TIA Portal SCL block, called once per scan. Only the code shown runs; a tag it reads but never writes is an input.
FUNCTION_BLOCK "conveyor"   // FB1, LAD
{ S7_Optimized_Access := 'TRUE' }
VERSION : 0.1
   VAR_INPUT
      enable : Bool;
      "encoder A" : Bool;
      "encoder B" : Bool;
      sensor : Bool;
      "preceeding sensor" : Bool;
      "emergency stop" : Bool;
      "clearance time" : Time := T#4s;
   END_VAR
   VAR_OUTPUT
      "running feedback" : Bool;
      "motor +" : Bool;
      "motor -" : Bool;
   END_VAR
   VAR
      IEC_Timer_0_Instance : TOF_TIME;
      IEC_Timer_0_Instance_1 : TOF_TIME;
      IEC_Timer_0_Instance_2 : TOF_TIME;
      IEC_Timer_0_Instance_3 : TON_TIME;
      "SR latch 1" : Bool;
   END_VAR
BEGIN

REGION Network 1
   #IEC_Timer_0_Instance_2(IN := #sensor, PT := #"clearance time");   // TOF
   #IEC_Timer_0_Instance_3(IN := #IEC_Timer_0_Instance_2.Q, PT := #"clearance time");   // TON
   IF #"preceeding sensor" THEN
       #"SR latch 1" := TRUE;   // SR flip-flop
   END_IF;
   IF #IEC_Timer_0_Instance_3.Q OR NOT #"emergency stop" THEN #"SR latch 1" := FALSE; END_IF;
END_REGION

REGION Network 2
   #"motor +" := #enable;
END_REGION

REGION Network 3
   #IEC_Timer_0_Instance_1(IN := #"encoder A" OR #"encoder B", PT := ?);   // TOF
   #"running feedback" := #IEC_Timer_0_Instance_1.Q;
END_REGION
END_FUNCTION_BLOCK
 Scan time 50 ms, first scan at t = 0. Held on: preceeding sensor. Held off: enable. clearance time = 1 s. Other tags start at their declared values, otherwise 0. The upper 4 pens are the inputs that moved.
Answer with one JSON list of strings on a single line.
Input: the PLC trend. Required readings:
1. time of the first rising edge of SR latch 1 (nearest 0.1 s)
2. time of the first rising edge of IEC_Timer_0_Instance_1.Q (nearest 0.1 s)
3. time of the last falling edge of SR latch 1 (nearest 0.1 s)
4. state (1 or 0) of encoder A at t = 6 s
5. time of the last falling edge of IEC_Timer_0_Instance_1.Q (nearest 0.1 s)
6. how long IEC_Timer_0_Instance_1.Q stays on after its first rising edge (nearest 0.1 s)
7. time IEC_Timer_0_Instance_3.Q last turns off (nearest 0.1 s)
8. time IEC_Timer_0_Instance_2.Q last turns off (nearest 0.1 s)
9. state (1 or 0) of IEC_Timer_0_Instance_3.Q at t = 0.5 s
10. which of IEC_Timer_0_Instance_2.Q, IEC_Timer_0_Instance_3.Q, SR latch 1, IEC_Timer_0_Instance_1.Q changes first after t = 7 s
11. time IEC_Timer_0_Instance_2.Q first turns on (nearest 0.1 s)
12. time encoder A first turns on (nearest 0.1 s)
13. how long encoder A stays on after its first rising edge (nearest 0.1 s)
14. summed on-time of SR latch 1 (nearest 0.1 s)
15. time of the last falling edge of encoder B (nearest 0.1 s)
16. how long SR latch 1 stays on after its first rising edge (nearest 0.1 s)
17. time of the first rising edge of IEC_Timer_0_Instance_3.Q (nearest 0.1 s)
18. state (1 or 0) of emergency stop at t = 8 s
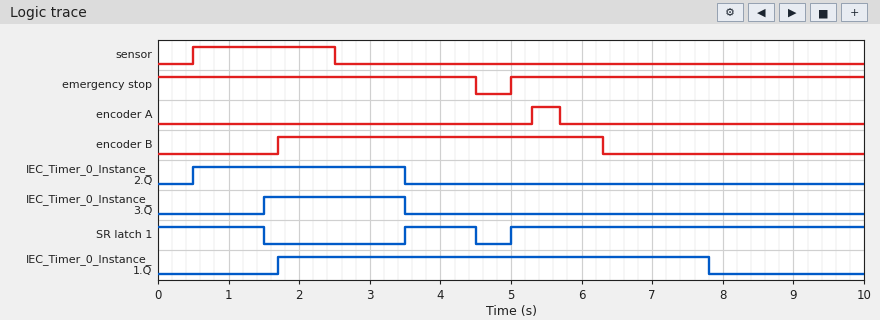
["3.5 s", "1.7 s", "4.5 s", "0", "7.8 s", "6.1 s", "3.5 s", "3.5 s", "0", "IEC_Timer_0_Instance_1.Q", "0.5 s", "5.3 s", "0.4 s", "7.5 s", "6.3 s", "1.0 s", "1.5 s", "1"]
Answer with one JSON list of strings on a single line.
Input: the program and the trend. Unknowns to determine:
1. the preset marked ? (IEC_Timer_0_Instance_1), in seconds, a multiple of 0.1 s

["1.5 s"]
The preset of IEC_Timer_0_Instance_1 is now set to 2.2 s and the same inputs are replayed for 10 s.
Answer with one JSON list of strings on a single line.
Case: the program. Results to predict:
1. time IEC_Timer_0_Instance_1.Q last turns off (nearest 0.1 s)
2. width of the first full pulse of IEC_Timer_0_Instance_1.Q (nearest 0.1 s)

["8.5 s", "6.8 s"]
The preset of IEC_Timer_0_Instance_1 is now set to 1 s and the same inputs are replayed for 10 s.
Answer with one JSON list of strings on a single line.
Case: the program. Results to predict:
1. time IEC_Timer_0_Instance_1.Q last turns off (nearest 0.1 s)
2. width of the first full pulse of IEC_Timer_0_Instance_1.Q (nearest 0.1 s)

["7.3 s", "5.6 s"]
